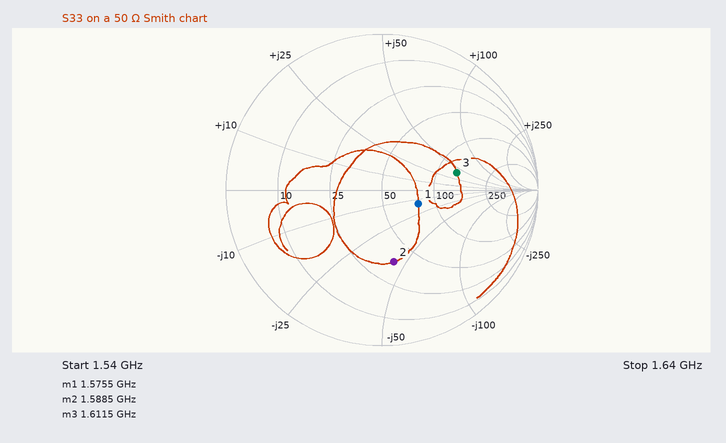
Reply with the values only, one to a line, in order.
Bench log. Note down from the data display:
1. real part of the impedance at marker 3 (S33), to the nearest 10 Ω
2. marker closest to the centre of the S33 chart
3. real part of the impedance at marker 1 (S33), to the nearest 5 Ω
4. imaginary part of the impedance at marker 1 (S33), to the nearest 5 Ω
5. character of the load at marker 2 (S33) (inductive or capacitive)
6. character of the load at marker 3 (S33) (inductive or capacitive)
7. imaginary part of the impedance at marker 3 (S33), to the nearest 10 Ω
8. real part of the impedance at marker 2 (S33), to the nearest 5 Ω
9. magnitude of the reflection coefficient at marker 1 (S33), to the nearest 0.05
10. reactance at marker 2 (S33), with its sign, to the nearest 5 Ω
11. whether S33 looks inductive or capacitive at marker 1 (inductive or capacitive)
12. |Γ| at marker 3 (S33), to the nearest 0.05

130 Ω
marker 1
80 Ω
-15 Ω
capacitive
inductive
+40 Ω
35 Ω
0.25
-45 Ω
capacitive
0.50
